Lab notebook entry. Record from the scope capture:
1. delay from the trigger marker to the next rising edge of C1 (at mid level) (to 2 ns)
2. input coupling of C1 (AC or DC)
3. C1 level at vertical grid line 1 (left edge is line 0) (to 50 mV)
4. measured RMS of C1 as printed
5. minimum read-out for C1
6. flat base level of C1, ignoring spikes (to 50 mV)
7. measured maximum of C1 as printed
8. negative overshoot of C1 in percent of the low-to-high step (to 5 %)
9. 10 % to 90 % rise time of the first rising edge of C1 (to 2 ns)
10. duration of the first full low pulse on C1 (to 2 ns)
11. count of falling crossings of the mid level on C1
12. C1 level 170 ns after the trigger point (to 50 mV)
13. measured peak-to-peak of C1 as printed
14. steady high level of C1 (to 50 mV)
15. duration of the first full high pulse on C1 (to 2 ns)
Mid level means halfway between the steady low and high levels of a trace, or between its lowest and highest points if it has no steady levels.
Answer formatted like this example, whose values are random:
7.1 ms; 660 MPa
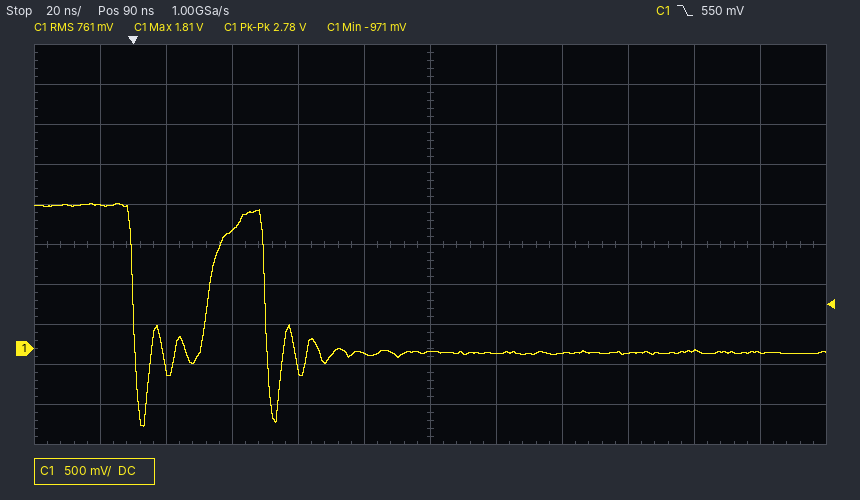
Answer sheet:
24 ns; DC; 1.80 V; 761 mV; -971 mV; -50 mV; 1.81 V; 50 %; 12 ns; 24 ns; 2; -50 mV; 2.78 V; 1.80 V; 16 ns
